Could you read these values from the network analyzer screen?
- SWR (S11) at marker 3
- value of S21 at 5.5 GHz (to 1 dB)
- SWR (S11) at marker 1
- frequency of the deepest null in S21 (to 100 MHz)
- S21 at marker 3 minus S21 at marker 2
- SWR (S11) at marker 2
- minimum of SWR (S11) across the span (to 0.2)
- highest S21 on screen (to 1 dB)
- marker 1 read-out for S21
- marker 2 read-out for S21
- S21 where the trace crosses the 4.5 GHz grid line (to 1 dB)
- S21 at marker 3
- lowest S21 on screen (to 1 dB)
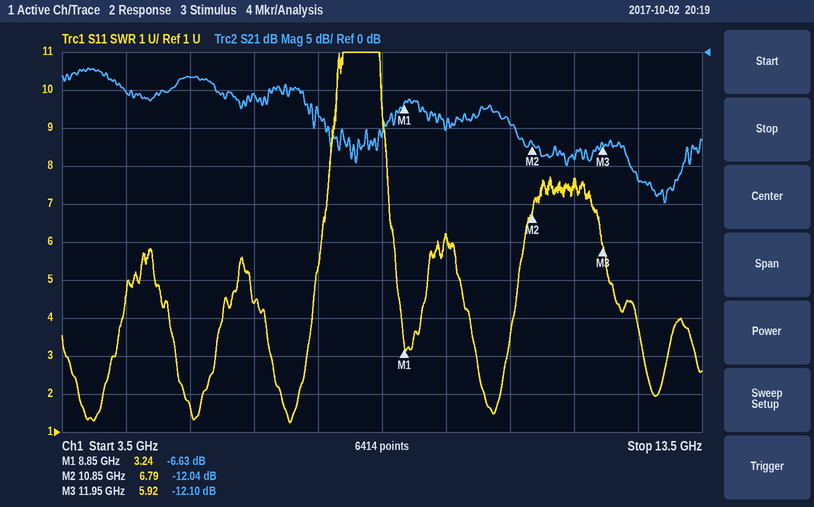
5.92
-3 dB
3.24
12.9 GHz
-0.06 dB
6.79
1.2
-2 dB
-6.63 dB
-12.04 dB
-5 dB
-12.10 dB
-20 dB
